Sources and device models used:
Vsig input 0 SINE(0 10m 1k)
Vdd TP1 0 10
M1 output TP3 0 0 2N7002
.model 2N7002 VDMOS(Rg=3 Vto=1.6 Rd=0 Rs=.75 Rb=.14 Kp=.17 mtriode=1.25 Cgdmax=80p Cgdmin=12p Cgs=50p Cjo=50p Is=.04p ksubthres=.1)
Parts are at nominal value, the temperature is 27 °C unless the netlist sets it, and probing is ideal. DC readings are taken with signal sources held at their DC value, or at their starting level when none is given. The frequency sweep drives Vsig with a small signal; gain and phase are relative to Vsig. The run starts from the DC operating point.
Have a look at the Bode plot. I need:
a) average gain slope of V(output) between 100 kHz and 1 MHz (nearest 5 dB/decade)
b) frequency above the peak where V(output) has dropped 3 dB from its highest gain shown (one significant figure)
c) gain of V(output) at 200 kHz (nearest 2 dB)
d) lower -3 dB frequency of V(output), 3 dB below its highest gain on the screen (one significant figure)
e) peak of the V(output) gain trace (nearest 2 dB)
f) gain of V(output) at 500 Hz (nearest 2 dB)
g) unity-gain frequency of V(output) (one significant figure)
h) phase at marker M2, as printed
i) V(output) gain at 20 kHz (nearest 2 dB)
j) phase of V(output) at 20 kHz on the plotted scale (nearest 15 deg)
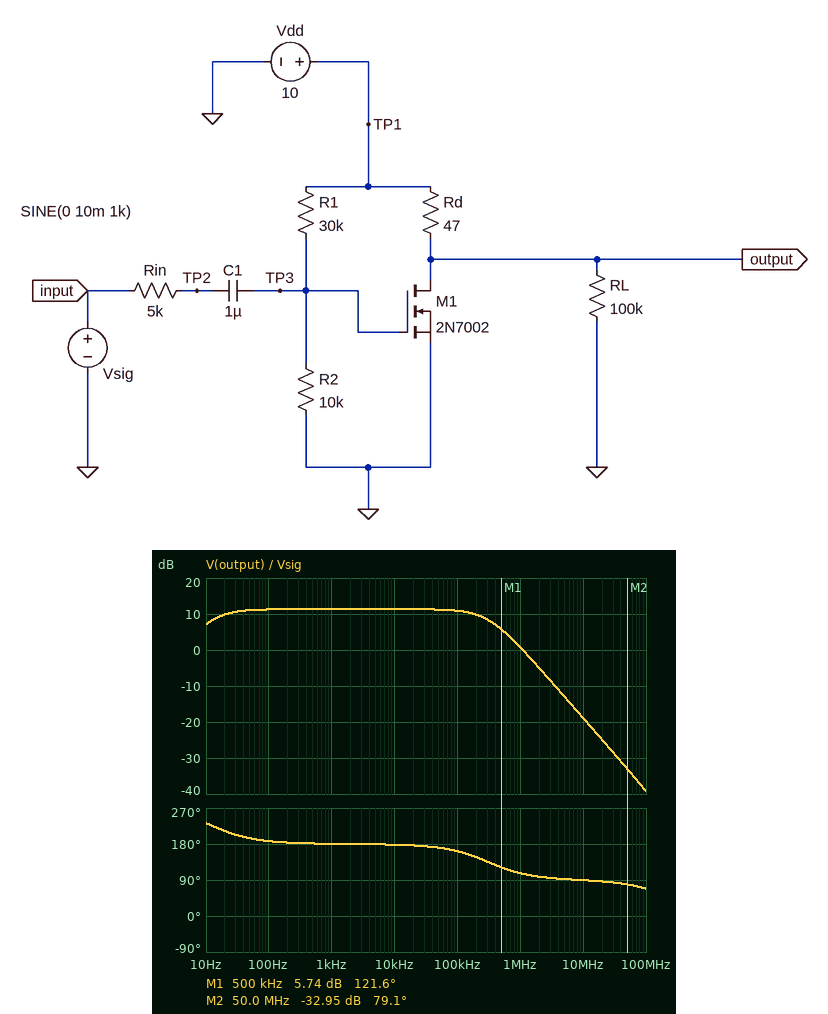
-10 dB/decade
300 kHz
10 dB
10 Hz
12 dB
12 dB
1 MHz
79.1 deg
12 dB
180 deg
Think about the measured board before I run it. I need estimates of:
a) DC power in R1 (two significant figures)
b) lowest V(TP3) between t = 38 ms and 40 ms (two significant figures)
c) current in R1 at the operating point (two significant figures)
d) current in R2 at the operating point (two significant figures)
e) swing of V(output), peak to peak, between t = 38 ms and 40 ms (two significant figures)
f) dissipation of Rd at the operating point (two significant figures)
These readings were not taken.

1.9 mW
2.5 V
250 µA
250 µA
74 mV
180 mW
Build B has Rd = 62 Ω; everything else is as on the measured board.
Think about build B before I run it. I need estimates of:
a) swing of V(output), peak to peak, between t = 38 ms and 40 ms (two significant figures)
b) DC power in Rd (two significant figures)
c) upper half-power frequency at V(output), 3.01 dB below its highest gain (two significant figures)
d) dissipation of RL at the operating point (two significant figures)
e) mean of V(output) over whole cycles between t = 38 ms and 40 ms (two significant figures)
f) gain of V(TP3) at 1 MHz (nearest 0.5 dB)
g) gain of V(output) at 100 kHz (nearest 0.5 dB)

97 mV
240 mW
240 kHz
380 µW
6.2 V
-17.0 dB
13.0 dB
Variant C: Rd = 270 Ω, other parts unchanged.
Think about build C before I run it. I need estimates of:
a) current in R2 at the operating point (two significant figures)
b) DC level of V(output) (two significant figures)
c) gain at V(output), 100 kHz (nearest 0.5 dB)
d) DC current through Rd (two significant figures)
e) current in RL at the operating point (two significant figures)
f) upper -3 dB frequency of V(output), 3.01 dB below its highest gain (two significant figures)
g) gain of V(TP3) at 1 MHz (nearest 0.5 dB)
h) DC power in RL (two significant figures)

250 µA
260 mV
-13.0 dB
36 mA
2.6 µA
330 kHz
-14.5 dB
680 nW
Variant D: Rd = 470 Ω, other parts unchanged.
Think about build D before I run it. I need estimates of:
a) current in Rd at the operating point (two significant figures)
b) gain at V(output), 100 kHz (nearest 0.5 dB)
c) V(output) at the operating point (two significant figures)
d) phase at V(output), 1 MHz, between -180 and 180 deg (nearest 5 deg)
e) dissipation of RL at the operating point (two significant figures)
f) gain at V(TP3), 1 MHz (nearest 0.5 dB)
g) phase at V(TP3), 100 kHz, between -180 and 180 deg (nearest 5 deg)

21 mA
-20.5 dB
140 mV
110 deg
190 nW
-13.5 dB
-15 deg
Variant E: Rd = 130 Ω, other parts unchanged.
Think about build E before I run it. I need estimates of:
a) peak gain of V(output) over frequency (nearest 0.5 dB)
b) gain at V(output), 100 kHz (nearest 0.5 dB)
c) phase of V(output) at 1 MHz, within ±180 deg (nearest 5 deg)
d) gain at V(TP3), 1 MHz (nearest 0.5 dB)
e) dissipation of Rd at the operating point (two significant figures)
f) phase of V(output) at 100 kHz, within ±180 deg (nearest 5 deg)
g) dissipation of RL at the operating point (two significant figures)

20.0 dB
12.0 dB
90 deg
-32.0 dB
500 mW
115 deg
38 µW
